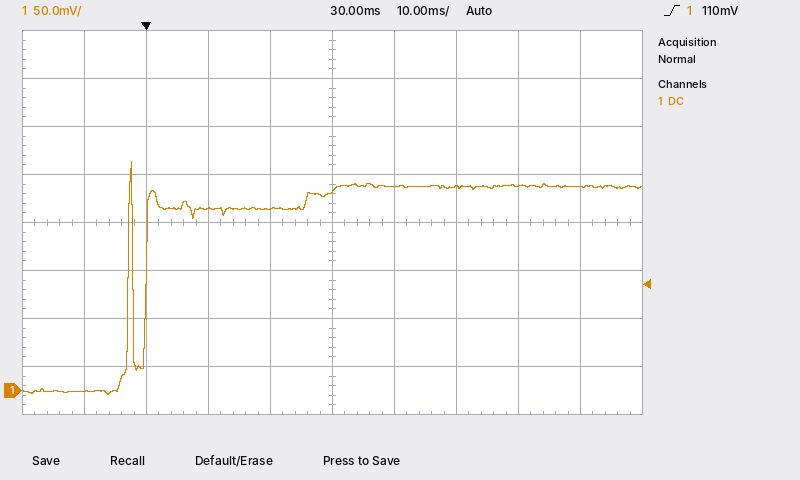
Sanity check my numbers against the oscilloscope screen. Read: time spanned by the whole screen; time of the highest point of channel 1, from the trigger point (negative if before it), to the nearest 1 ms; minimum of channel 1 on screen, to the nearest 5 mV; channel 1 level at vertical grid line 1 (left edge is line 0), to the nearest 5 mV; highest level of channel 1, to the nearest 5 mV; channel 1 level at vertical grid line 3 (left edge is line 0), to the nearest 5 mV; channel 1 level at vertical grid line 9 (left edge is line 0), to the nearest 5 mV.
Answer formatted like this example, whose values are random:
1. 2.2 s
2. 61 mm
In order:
1. 100 ms
2. -2 ms
3. -5 mV
4. 0 mV
5. 240 mV
6. 190 mV
7. 210 mV
